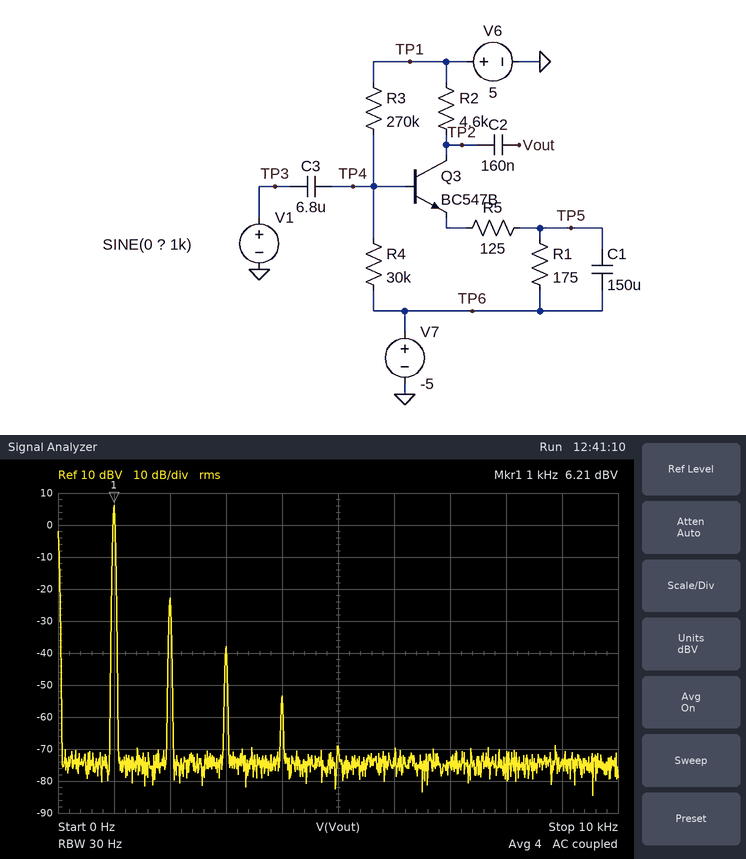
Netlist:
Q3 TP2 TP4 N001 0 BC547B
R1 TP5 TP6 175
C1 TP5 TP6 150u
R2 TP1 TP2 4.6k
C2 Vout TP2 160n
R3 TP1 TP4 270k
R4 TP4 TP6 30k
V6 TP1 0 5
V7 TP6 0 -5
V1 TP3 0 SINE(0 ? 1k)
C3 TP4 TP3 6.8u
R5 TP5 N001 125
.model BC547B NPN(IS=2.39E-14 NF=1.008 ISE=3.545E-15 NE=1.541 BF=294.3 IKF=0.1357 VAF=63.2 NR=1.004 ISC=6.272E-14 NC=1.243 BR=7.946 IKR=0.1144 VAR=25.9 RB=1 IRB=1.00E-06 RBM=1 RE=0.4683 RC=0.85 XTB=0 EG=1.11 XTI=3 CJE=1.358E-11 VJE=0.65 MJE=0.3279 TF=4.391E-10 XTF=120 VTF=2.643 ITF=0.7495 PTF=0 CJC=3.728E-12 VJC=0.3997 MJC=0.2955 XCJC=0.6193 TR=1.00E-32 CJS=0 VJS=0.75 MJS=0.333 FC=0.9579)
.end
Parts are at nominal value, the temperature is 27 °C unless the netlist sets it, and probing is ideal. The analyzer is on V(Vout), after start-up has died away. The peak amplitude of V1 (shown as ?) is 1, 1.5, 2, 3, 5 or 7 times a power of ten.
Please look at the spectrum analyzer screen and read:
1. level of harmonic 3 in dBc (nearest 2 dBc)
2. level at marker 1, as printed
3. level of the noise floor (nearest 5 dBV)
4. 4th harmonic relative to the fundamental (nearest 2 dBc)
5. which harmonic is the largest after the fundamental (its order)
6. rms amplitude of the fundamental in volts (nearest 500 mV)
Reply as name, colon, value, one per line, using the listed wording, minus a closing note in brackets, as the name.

level of harmonic 3 in dBc: -44 dBc
level at marker 1, as printed: 6.21 dBV
level of the noise floor: -75 dBV
4th harmonic relative to the fundamental: -60 dBc
which harmonic is the largest after the fundamental: 2
rms amplitude of the fundamental in volts: 2.0 V
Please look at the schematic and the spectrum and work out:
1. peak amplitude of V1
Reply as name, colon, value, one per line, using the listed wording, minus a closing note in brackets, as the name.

peak amplitude of V1: 100 mV
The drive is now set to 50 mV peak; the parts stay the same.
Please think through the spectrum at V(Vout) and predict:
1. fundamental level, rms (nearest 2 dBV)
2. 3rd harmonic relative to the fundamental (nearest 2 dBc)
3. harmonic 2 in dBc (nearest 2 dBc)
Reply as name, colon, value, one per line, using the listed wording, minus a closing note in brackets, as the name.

fundamental level, rms: 0 dBV
3rd harmonic relative to the fundamental: -58 dBc
harmonic 2 in dBc: -36 dBc
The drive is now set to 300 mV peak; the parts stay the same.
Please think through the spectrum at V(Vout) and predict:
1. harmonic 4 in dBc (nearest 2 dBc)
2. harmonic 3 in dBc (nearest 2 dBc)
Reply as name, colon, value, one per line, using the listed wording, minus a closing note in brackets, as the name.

harmonic 4 in dBc: -24 dBc
harmonic 3 in dBc: -30 dBc
